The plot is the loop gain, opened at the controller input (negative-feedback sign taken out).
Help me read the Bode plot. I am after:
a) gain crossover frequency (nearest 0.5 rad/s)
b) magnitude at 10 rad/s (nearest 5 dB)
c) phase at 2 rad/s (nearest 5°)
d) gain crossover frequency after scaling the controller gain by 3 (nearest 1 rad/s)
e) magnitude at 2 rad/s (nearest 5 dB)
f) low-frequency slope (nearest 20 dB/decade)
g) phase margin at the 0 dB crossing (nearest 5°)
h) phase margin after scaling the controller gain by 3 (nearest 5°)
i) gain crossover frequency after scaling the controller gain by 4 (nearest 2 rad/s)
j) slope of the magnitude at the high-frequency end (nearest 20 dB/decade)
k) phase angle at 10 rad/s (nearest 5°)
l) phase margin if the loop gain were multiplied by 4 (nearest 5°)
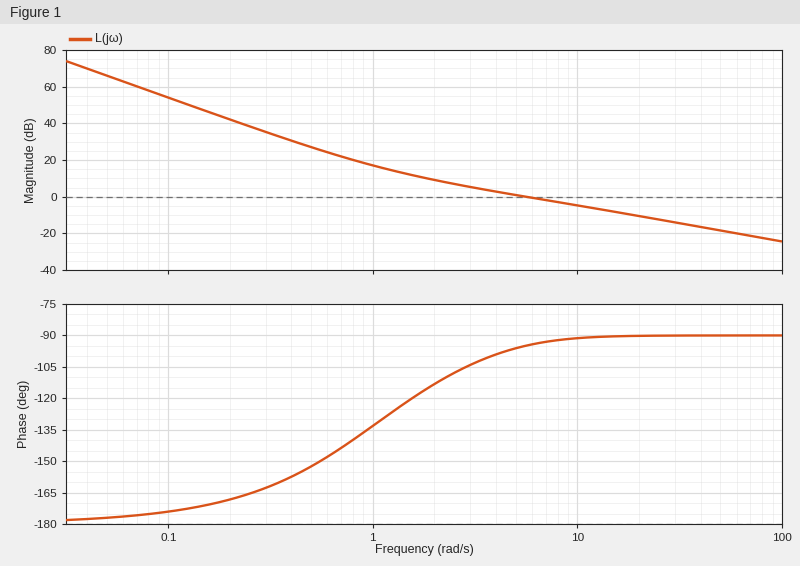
5.5 rad/s
-5 dB
-115°
18 rad/s
10 dB
-40 dB/decade
85°
90°
24 rad/s
-20 dB/decade
-90°
90°
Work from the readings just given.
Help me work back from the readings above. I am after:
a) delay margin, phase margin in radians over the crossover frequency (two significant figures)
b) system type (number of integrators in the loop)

0.27 s
2
